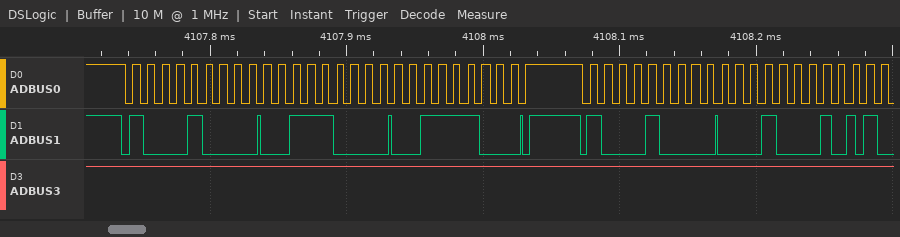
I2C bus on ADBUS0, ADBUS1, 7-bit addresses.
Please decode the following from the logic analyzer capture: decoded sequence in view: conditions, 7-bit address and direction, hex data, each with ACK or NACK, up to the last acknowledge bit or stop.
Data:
start, address 44 write ACK, 38 ACK, 3C ACK, stop, start, address 44 write ACK, 11 ACK
